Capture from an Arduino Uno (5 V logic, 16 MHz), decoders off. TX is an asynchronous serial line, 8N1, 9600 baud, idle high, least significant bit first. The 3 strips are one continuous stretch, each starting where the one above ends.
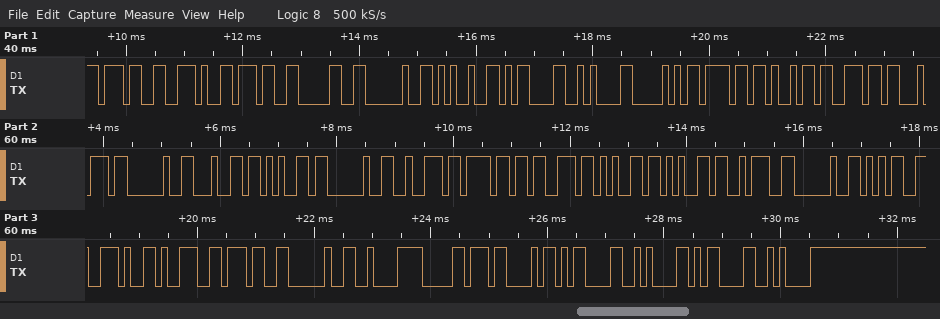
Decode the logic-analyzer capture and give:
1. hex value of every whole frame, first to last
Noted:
37 2E 37 30 20 25 0D 0A 50 6F 69 6E 74 20 64 65 20 72 6F 73 65 65 3A 20 35 2E 39 37 20 C2 B0 43 0D 0A 0D 0A
